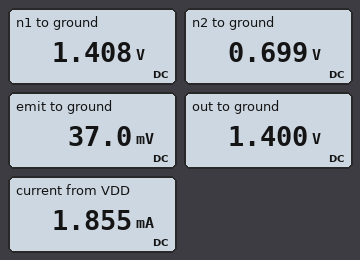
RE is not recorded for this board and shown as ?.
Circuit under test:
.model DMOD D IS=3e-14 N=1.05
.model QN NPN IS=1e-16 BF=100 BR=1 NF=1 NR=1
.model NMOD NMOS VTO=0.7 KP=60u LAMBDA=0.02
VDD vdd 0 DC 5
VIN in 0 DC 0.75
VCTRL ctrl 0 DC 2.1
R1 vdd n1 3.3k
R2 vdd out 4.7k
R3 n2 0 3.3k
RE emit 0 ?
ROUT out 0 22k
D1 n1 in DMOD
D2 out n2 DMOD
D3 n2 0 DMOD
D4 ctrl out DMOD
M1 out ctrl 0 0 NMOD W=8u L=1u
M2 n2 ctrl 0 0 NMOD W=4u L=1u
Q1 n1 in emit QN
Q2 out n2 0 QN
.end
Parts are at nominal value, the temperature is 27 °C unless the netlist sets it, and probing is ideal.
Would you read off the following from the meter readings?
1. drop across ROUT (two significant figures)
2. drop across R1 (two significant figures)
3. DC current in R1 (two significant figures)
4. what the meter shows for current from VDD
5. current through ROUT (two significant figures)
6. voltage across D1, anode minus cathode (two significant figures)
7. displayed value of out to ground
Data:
1.4 V
3.6 V
1.1 mA
1.855 mA
64 µA
660 mV
1.400 V
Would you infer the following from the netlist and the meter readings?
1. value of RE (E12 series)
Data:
390 Ω
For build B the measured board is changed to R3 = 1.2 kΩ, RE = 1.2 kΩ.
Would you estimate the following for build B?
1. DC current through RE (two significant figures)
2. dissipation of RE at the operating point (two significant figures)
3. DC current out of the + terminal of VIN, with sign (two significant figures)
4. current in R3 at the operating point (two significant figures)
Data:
46 µA
2.6 µW
-1.0 mA
580 µA
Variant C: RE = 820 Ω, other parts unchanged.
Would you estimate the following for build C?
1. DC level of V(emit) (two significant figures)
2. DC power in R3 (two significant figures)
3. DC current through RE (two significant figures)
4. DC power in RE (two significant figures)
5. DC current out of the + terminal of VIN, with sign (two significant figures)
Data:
49 mV
150 µW
60 µA
2.9 µW
-1.0 mA
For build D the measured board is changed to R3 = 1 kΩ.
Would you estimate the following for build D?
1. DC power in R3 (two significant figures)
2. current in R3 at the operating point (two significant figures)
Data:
490 µW
700 µA
